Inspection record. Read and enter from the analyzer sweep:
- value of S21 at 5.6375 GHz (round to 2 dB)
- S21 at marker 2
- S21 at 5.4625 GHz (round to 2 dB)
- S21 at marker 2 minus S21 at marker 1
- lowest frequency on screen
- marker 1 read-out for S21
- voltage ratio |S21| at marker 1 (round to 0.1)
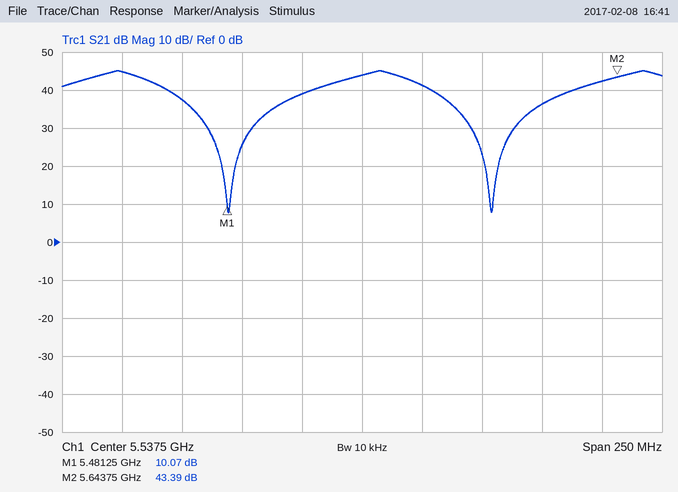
42 dB
43.39 dB
38 dB
33.32 dB
5.4125 GHz
10.07 dB
3.2
